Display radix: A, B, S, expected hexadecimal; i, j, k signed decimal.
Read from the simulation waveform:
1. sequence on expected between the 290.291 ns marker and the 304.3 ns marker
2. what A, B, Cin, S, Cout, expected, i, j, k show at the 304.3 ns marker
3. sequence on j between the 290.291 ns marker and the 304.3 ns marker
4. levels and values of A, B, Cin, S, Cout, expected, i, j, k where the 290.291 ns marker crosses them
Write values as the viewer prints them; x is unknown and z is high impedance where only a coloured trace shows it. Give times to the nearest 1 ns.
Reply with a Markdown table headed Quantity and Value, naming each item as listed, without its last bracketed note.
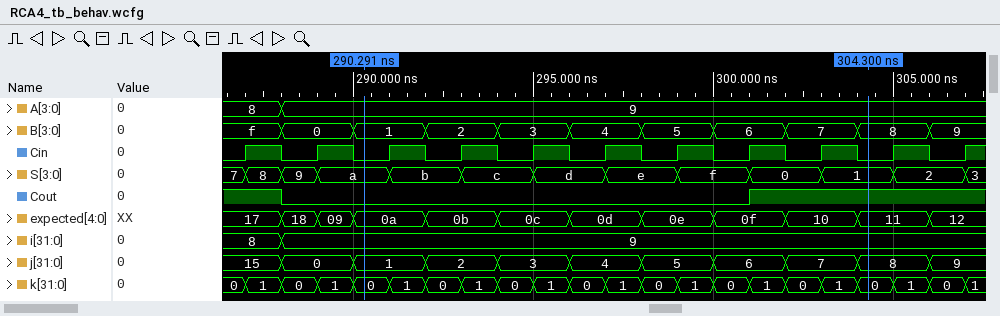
| Quantity | Value |
|---|---|
| sequence on expected between the 290.291 ns marker and the 304.3 ns marker | 0a, 0b, 0c, 0d, 0e, 0f, 10, 11 |
| what A, B, Cin, S, Cout, expected, i, j, k show at the 304.3 ns marker | A=9, B=8, Cin=0, S=1, Cout=1, expected=11, i=9, j=8, k=0 |
| sequence on j between the 290.291 ns marker and the 304.3 ns marker | 1, 2, 3, 4, 5, 6, 7, 8 |
| levels and values of A, B, Cin, S, Cout, expected, i, j, k where the 290.291 ns marker crosses them | A=9, B=1, Cin=0, S=a, Cout=0, expected=0a, i=9, j=1, k=0 |
